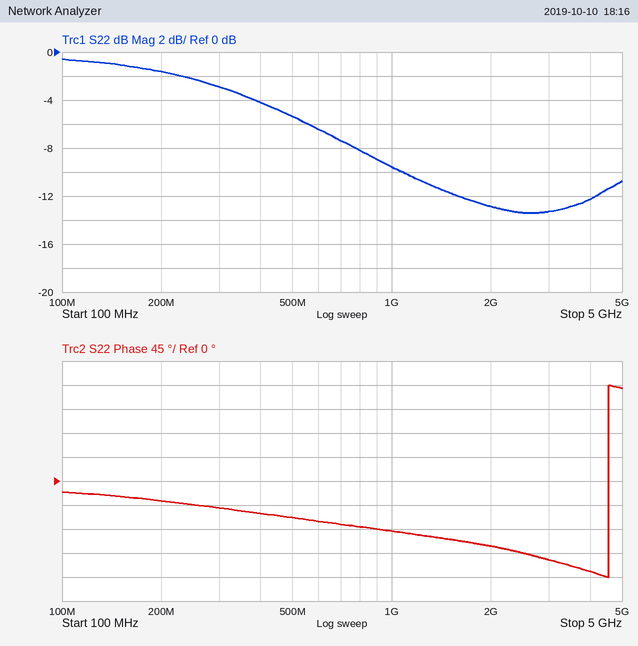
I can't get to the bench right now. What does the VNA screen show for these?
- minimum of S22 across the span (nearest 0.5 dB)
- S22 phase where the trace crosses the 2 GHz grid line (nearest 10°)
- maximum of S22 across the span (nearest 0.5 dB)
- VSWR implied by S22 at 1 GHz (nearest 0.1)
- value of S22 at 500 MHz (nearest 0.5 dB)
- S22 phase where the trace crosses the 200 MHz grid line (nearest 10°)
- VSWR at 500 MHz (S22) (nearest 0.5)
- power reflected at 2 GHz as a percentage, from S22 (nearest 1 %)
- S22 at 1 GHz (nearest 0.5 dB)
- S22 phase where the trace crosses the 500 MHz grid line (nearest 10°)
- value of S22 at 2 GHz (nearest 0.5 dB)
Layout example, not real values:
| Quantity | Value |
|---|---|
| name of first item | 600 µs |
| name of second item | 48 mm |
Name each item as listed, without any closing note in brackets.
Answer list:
| Quantity | Value |
|---|---|
| minimum of S22 across the span | -13.5 dB |
| S22 phase where the trace crosses the 2 GHz grid line | -120° |
| maximum of S22 across the span | -0.5 dB |
| VSWR implied by S22 at 1 GHz | 2.0 |
| value of S22 at 500 MHz | -5.5 dB |
| S22 phase where the trace crosses the 200 MHz grid line | -40° |
| VSWR at 500 MHz (S22) | 3.5 |
| power reflected at 2 GHz as a percentage, from S22 | 5 % |
| S22 at 1 GHz | -9.5 dB |
| S22 phase where the trace crosses the 500 MHz grid line | -70° |
| value of S22 at 2 GHz | -13.0 dB |
